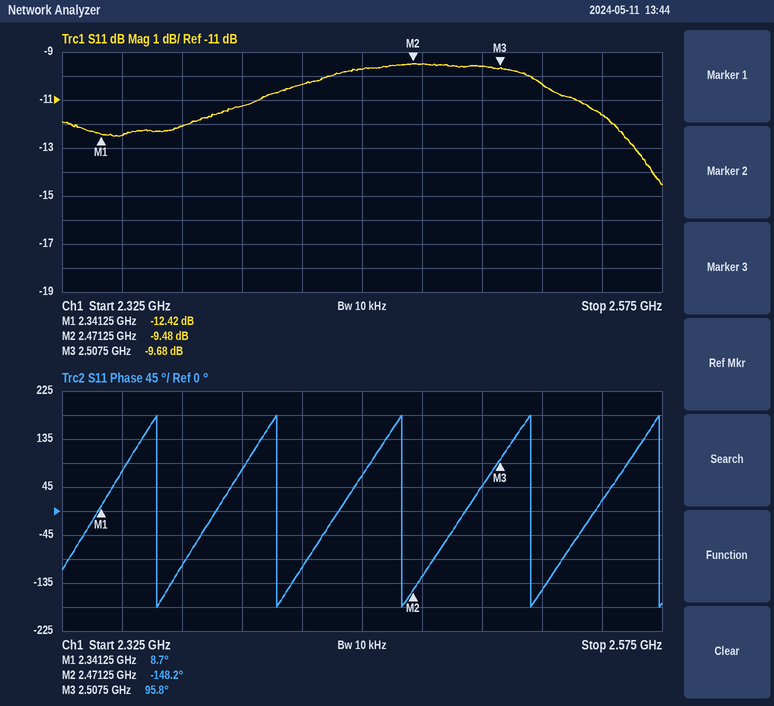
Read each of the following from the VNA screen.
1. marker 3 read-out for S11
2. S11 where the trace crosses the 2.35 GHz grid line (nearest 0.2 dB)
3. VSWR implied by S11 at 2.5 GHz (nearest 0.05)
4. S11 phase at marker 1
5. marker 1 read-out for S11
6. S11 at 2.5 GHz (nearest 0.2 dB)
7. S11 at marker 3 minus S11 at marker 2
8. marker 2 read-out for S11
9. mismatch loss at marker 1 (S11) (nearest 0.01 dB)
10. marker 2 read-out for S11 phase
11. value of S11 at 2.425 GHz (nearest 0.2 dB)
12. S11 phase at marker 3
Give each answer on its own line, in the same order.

-9.68 dB
-12.4 dB
2.00
8.7°
-12.42 dB
-9.6 dB
-0.20 dB
-9.48 dB
0.26 dB
-148.2°
-10.4 dB
95.8°
